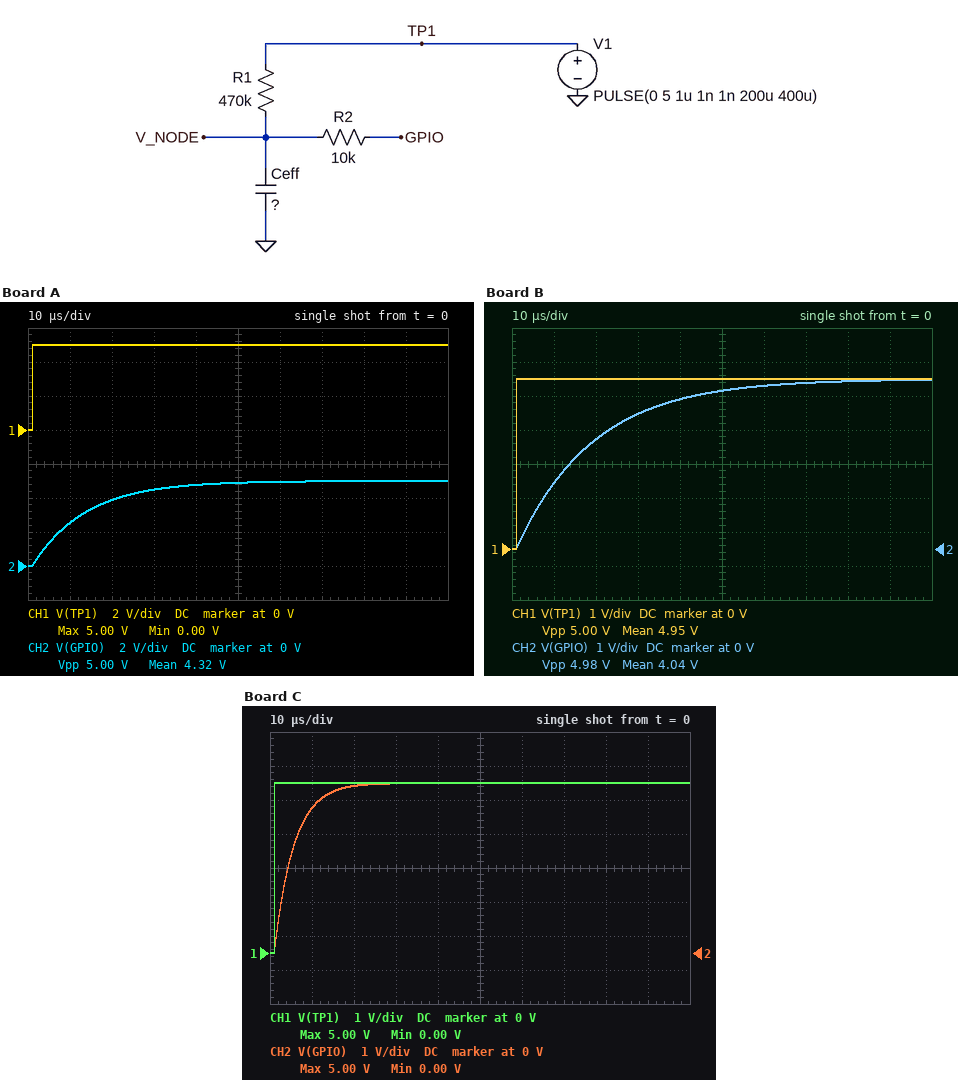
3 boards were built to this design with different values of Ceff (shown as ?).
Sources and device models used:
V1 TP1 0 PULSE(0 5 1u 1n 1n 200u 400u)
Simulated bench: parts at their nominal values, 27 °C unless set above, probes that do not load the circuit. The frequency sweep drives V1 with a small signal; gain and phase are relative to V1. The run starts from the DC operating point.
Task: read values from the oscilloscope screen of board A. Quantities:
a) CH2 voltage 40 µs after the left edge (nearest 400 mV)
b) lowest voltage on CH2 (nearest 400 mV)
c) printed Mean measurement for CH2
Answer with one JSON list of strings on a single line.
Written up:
["4.8 V", "0 V", "4.32 V"]
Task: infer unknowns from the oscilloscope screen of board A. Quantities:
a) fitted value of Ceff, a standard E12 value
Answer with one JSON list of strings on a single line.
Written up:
["27 pF"]
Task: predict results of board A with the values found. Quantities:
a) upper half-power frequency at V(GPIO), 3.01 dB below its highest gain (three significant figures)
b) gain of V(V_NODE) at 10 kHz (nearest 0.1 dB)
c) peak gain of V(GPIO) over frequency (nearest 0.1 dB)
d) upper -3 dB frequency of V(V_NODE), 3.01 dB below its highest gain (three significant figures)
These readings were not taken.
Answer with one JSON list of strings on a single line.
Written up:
["12.5 kHz", "-2.1 dB", "0 dB", "12.5 kHz"]
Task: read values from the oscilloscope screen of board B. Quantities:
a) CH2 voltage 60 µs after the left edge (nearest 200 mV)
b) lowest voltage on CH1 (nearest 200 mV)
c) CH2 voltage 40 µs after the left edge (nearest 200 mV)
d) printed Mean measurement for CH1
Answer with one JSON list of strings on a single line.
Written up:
["4.8 V", "0 V", "4.4 V", "4.95 V"]
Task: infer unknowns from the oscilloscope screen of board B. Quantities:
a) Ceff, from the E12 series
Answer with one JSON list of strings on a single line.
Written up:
["39 pF"]
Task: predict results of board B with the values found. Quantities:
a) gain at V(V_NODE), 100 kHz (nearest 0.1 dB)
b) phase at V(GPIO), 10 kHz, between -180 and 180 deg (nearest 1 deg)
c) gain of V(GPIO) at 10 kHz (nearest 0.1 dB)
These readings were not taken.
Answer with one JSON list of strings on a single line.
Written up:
["-21.3 dB", "-49 deg", "-3.7 dB"]
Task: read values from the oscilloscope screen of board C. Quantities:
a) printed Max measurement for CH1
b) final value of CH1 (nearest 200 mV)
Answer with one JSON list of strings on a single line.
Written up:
["5.00 V", "5.0 V"]
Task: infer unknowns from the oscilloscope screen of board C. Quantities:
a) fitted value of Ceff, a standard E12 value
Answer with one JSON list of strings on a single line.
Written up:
["10 pF"]
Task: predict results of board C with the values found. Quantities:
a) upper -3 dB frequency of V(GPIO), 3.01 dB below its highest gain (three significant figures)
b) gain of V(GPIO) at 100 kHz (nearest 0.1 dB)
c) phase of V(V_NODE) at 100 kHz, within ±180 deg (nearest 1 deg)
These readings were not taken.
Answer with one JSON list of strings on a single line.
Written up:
["33.9 kHz", "-9.9 dB", "-71 deg"]
